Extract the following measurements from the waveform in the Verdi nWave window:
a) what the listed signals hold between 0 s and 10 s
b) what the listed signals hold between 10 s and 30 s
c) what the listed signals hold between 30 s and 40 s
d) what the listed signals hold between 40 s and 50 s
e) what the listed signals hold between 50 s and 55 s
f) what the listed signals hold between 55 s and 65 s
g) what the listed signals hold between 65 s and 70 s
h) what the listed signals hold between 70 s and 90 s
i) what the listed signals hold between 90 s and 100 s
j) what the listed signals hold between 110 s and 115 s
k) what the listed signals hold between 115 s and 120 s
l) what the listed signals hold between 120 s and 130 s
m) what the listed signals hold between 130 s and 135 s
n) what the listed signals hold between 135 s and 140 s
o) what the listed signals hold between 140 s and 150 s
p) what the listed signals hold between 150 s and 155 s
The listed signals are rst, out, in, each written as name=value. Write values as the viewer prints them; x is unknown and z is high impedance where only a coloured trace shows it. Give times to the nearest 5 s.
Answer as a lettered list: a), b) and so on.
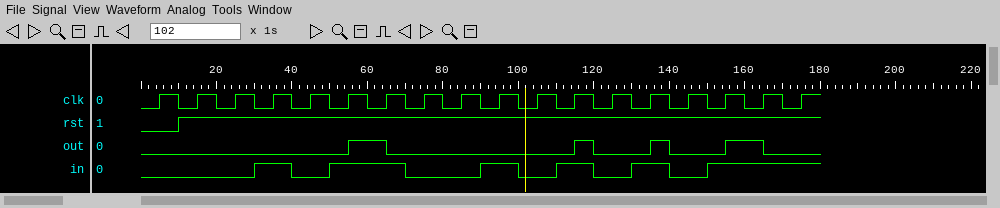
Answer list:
a) rst=0, out=0, in=0
b) rst=1, out=0, in=0
c) rst=1, out=0, in=1
d) rst=1, out=0, in=0
e) rst=1, out=0, in=1
f) rst=1, out=1, in=1
g) rst=1, out=0, in=1
h) rst=1, out=0, in=0
i) rst=1, out=0, in=1
j) rst=1, out=0, in=1
k) rst=1, out=1, in=1
l) rst=1, out=0, in=0
m) rst=1, out=0, in=1
n) rst=1, out=1, in=1
o) rst=1, out=0, in=0
p) rst=1, out=0, in=1
